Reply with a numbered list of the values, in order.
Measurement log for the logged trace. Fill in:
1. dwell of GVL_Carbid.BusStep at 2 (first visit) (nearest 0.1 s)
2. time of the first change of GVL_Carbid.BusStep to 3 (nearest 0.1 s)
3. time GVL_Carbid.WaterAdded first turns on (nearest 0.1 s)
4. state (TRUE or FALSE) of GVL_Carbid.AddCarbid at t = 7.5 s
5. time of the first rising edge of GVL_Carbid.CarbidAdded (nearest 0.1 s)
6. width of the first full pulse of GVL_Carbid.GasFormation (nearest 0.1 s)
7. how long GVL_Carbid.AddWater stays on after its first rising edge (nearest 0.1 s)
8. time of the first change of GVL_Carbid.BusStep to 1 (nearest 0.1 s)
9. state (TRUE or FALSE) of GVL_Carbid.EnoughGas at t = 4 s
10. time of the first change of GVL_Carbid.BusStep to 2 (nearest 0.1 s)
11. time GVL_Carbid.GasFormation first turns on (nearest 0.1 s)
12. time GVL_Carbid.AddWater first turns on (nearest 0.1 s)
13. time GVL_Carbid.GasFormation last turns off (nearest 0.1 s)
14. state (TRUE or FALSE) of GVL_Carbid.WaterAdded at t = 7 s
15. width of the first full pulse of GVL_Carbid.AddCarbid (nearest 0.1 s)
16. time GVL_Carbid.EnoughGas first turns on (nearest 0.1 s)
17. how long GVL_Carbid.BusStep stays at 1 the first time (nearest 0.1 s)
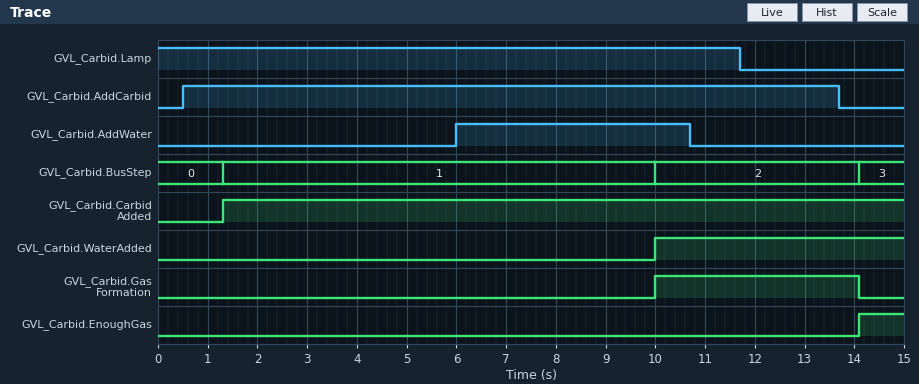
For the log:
1. 4.1 s
2. 14.1 s
3. 10.0 s
4. TRUE
5. 1.3 s
6. 4.1 s
7. 4.7 s
8. 1.3 s
9. FALSE
10. 10.0 s
11. 10.0 s
12. 6.0 s
13. 14.1 s
14. FALSE
15. 13.2 s
16. 14.1 s
17. 8.7 s
